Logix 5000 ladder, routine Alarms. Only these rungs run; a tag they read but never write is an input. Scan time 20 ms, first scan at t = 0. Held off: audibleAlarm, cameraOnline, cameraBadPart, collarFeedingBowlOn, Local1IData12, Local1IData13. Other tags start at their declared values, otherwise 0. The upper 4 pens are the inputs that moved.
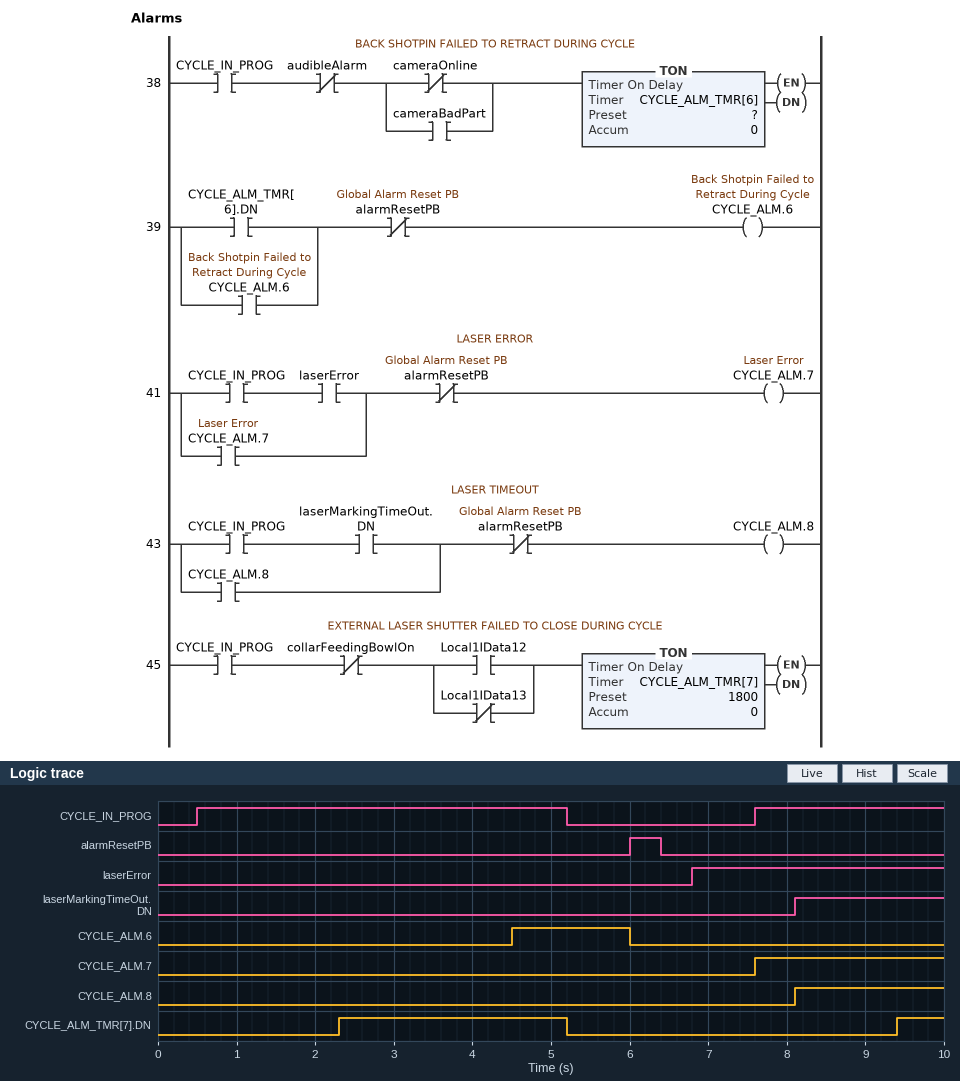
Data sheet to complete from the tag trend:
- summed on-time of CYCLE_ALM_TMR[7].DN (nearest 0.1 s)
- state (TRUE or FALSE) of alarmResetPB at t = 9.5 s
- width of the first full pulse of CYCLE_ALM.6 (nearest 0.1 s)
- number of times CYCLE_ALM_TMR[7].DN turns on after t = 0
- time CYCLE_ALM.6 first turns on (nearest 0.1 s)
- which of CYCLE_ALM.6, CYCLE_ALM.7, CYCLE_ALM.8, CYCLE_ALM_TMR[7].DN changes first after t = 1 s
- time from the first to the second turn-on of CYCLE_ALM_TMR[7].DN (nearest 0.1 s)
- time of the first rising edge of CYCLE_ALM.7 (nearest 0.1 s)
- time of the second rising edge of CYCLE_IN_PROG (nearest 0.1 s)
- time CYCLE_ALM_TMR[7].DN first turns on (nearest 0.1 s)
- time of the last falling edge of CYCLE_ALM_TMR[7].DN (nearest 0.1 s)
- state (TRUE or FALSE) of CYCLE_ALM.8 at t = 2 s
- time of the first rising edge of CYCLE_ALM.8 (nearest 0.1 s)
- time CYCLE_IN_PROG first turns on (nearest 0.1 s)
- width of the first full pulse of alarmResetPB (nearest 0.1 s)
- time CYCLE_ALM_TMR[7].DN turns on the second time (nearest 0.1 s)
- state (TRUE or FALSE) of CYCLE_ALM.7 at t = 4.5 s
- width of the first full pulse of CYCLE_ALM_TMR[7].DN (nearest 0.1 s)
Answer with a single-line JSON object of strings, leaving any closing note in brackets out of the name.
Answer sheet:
{"summed on-time of CYCLE_ALM_TMR[7].DN": "3.5 s", "state (TRUE or FALSE) of alarmResetPB at t = 9.5 s": "FALSE", "width of the first full pulse of CYCLE_ALM.6": "1.5 s", "number of times CYCLE_ALM_TMR[7].DN turns on after t = 0": "2", "time CYCLE_ALM.6 first turns on": "4.5 s", "which of CYCLE_ALM.6, CYCLE_ALM.7, CYCLE_ALM.8, CYCLE_ALM_TMR[7].DN changes first after t = 1 s": "CYCLE_ALM_TMR[7].DN", "time from the first to the second turn-on of CYCLE_ALM_TMR[7].DN": "7.1 s", "time of the first rising edge of CYCLE_ALM.7": "7.6 s", "time of the second rising edge of CYCLE_IN_PROG": "7.6 s", "time CYCLE_ALM_TMR[7].DN first turns on": "2.3 s", "time of the last falling edge of CYCLE_ALM_TMR[7].DN": "5.2 s", "state (TRUE or FALSE) of CYCLE_ALM.8 at t = 2 s": "FALSE", "time of the first rising edge of CYCLE_ALM.8": "8.1 s", "time CYCLE_IN_PROG first turns on": "0.5 s", "width of the first full pulse of alarmResetPB": "0.4 s", "time CYCLE_ALM_TMR[7].DN turns on the second time": "9.4 s", "state (TRUE or FALSE) of CYCLE_ALM.7 at t = 4.5 s": "FALSE", "width of the first full pulse of CYCLE_ALM_TMR[7].DN": "2.9 s"}
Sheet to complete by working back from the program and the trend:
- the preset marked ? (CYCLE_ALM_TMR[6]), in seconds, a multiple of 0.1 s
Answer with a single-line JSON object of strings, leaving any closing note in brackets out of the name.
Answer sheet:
{"the preset marked ? (CYCLE_ALM_TMR[6]), in seconds, a multiple of 0.1 s": "4.0 s"}
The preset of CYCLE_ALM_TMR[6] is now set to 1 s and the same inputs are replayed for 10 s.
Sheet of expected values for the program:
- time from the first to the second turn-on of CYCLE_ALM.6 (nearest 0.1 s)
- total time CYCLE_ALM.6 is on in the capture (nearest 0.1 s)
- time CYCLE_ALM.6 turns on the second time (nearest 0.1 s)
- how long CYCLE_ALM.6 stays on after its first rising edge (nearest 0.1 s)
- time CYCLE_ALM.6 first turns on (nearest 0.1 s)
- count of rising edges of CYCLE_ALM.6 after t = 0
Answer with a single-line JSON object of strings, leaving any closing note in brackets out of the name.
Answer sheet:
{"time from the first to the second turn-on of CYCLE_ALM.6": "7.1 s", "total time CYCLE_ALM.6 is on in the capture": "5.9 s", "time CYCLE_ALM.6 turns on the second time": "8.6 s", "how long CYCLE_ALM.6 stays on after its first rising edge": "4.5 s", "time CYCLE_ALM.6 first turns on": "1.5 s", "count of rising edges of CYCLE_ALM.6 after t = 0": "2"}
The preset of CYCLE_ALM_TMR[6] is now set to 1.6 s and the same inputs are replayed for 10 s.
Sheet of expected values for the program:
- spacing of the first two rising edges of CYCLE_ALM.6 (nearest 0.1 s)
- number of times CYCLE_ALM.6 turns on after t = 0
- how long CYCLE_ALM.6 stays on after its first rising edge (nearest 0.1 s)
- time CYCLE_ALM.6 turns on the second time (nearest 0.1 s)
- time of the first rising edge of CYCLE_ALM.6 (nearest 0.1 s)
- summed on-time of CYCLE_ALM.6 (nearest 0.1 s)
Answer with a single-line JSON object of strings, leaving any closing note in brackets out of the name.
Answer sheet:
{"spacing of the first two rising edges of CYCLE_ALM.6": "7.1 s", "number of times CYCLE_ALM.6 turns on after t = 0": "2", "how long CYCLE_ALM.6 stays on after its first rising edge": "3.9 s", "time CYCLE_ALM.6 turns on the second time": "9.2 s", "time of the first rising edge of CYCLE_ALM.6": "2.1 s", "summed on-time of CYCLE_ALM.6": "4.7 s"}
